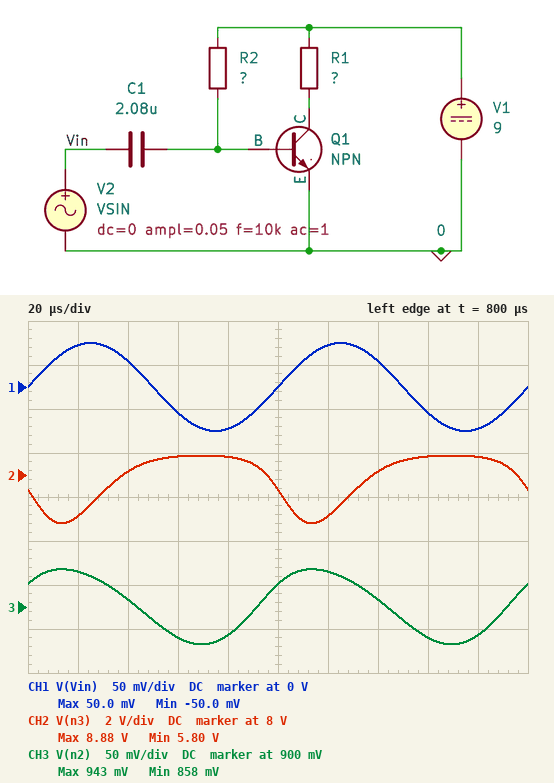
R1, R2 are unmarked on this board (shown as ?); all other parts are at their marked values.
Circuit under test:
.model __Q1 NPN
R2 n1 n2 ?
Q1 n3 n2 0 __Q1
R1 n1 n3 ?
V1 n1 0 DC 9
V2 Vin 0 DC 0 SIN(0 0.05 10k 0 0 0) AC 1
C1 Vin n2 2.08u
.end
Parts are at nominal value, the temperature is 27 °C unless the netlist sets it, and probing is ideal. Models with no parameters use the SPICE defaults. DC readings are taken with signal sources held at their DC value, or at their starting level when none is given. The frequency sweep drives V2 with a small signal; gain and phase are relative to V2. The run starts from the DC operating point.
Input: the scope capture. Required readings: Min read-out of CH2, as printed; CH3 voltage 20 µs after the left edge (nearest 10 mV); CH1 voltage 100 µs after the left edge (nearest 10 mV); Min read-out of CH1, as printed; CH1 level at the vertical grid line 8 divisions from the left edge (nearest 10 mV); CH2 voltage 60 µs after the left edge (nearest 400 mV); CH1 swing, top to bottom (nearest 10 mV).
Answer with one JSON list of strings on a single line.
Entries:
["5.80 V", "940 mV", "0 V", "-50.0 mV", "-30 mV", "8.8 V", "100 mV"]
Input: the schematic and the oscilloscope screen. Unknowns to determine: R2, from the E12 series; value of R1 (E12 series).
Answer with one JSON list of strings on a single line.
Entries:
["3.3 kΩ", "4.7 Ω"]
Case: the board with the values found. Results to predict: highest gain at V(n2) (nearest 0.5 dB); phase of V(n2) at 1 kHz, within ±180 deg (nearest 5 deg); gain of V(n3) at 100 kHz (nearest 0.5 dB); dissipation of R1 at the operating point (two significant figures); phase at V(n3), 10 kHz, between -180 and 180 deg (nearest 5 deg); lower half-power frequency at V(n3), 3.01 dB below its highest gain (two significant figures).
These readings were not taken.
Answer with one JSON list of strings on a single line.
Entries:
["0 dB", "80 deg", "33.0 dB", "280 mW", "-145 deg", "7.3 kHz"]
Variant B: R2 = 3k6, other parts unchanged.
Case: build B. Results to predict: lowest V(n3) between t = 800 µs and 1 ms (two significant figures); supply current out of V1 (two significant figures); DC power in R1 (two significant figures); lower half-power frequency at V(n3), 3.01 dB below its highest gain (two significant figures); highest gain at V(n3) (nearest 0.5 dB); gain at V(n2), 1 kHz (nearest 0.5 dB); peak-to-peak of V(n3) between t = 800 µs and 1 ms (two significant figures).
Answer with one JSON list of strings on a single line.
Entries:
["6.0 V", "230 mA", "240 mW", "6.7 kHz", "32.0 dB", "-16.5 dB", "2.9 V"]
